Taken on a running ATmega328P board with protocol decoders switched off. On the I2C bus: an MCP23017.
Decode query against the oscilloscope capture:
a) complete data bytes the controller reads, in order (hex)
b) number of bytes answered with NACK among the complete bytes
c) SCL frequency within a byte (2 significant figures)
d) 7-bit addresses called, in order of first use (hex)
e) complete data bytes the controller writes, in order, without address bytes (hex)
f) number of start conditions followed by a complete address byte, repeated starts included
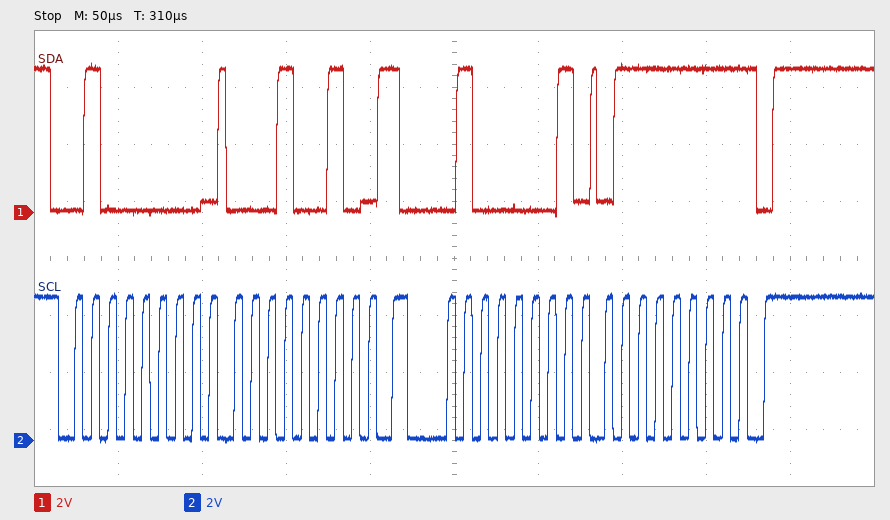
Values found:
7F
1
100 kHz
0x20
12
2
